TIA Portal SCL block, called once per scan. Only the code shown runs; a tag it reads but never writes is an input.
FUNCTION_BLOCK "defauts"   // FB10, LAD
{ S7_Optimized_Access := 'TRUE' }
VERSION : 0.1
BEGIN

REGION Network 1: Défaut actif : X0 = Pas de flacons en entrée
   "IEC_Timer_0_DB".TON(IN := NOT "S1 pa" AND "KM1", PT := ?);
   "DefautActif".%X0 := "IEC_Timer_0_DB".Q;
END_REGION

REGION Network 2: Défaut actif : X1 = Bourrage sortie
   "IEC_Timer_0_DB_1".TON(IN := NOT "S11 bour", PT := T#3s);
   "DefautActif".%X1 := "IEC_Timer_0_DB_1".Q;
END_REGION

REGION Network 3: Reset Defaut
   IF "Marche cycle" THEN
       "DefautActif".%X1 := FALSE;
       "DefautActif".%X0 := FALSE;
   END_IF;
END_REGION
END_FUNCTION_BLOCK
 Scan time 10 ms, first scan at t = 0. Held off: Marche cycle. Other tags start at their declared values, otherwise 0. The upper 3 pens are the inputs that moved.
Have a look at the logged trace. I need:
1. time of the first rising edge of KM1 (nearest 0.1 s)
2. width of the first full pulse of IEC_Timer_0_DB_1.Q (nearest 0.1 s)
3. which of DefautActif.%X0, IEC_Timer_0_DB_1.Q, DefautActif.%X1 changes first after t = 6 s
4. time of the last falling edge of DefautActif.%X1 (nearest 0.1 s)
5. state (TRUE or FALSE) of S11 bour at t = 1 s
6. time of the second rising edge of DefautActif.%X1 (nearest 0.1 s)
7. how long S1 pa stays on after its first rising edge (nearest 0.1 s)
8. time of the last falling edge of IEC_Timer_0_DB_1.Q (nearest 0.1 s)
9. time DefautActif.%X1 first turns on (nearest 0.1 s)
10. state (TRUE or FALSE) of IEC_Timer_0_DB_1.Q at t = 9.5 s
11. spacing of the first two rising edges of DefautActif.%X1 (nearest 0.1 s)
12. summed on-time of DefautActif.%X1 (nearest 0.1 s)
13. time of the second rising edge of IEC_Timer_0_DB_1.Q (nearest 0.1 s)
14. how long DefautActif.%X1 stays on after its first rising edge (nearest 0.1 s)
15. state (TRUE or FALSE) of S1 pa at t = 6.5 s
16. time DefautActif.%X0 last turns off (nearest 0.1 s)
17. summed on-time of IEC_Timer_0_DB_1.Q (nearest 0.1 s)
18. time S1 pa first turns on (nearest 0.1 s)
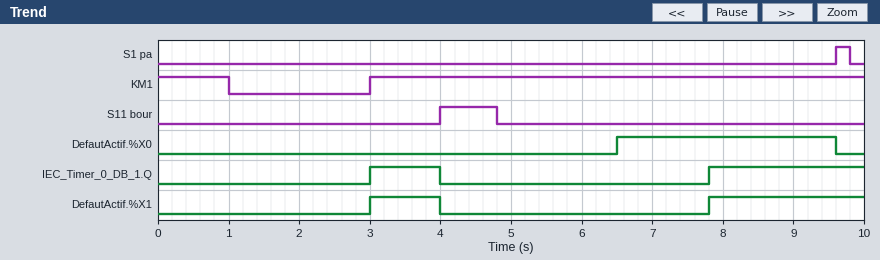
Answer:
3.0 s
1.0 s
DefautActif.%X0
4.0 s
FALSE
7.8 s
0.2 s
4.0 s
3.0 s
TRUE
4.8 s
3.2 s
7.8 s
1.0 s
FALSE
9.6 s
3.2 s
9.6 s
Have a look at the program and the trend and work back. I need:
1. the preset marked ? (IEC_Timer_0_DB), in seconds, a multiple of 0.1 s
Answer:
3.5 s
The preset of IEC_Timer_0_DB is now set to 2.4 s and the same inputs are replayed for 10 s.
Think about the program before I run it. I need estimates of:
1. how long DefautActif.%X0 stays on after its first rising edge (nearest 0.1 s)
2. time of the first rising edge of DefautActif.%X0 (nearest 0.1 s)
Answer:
4.2 s
5.4 s
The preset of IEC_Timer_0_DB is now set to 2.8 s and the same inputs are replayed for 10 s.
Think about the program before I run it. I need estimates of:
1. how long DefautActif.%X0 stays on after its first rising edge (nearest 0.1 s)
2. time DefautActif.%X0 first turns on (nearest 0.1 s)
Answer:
3.8 s
5.8 s
